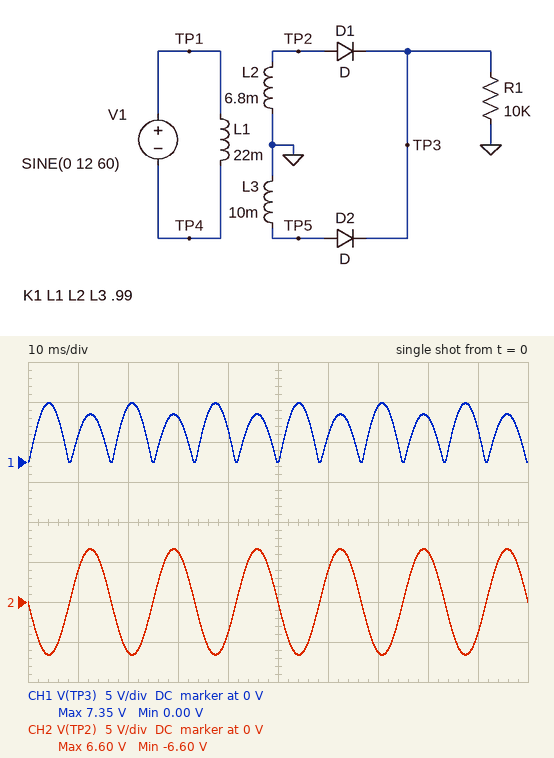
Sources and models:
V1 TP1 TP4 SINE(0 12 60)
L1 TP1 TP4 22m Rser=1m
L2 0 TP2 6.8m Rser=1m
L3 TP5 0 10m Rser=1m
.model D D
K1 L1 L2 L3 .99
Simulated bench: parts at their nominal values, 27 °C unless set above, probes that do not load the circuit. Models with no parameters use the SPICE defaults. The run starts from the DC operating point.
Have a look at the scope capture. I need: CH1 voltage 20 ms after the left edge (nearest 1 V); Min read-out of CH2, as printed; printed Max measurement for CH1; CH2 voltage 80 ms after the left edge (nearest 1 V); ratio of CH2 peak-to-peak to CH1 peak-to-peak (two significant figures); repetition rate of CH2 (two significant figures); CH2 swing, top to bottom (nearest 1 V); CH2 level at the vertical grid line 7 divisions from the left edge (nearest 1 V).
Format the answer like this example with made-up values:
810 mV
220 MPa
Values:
7 V
-6.60 V
7.35 V
6 V
1.8
60 Hz
13 V
-6 V
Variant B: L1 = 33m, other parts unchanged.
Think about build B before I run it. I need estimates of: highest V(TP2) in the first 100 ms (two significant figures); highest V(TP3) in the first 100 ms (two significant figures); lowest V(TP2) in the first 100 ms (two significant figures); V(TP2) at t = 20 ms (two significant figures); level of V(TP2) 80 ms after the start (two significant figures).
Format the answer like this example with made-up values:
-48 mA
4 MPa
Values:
5.4 V
5.9 V
-5.4 V
-5.1 V
5.1 V
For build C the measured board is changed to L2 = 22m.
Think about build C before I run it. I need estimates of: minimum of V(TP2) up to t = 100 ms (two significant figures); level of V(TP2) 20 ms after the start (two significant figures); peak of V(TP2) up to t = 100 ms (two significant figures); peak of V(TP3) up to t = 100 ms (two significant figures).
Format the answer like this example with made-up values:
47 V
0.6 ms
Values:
-12 V
-11 V
12 V
11 V
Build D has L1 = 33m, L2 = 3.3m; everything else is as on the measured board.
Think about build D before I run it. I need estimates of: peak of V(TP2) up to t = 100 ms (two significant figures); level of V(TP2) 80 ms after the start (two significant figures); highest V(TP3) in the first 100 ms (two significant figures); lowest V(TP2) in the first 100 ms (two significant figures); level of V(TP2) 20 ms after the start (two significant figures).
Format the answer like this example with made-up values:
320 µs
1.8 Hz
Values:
3.8 V
3.6 V
5.9 V
-3.8 V
-3.6 V
